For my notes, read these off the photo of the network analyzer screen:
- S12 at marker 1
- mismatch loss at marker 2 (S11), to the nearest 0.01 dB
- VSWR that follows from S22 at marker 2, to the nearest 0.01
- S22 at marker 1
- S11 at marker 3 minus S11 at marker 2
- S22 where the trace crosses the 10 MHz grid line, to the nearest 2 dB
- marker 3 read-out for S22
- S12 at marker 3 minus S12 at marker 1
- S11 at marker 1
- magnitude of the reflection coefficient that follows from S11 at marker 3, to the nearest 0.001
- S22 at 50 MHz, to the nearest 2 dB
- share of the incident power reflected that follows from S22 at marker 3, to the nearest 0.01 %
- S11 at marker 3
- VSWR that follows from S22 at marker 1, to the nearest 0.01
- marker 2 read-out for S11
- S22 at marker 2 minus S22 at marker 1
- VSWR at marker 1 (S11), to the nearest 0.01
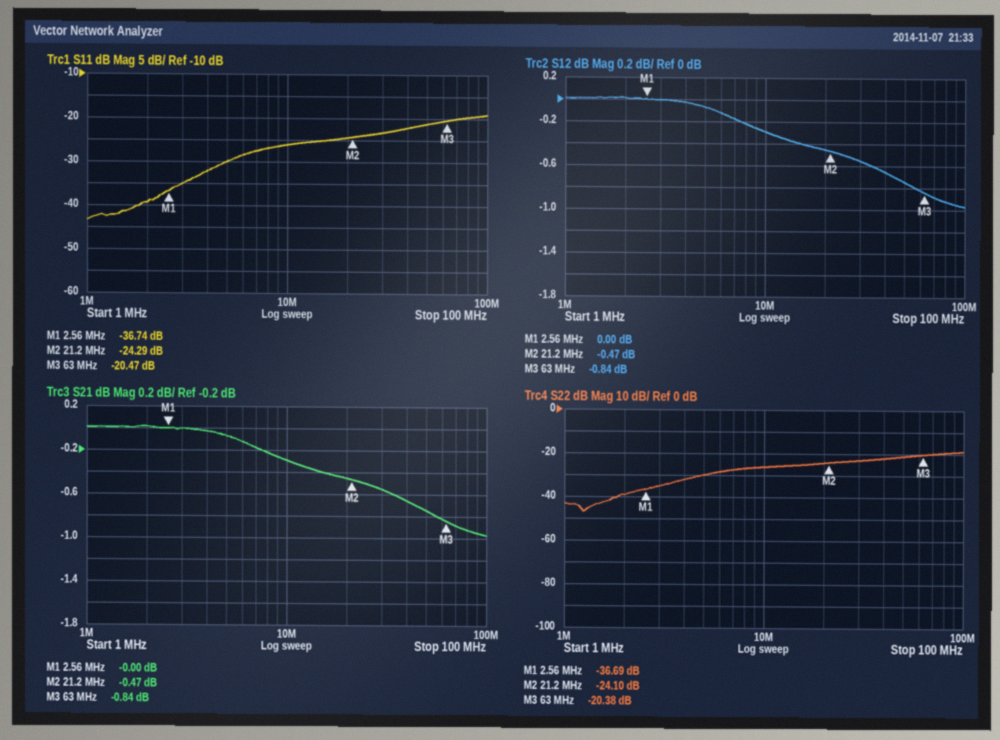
0.00 dB
0.02 dB
1.13
-36.69 dB
3.82 dB
-26 dB
-20.38 dB
-0.84 dB
-36.74 dB
0.095
-22 dB
0.92 %
-20.47 dB
1.03
-24.29 dB
12.59 dB
1.03
